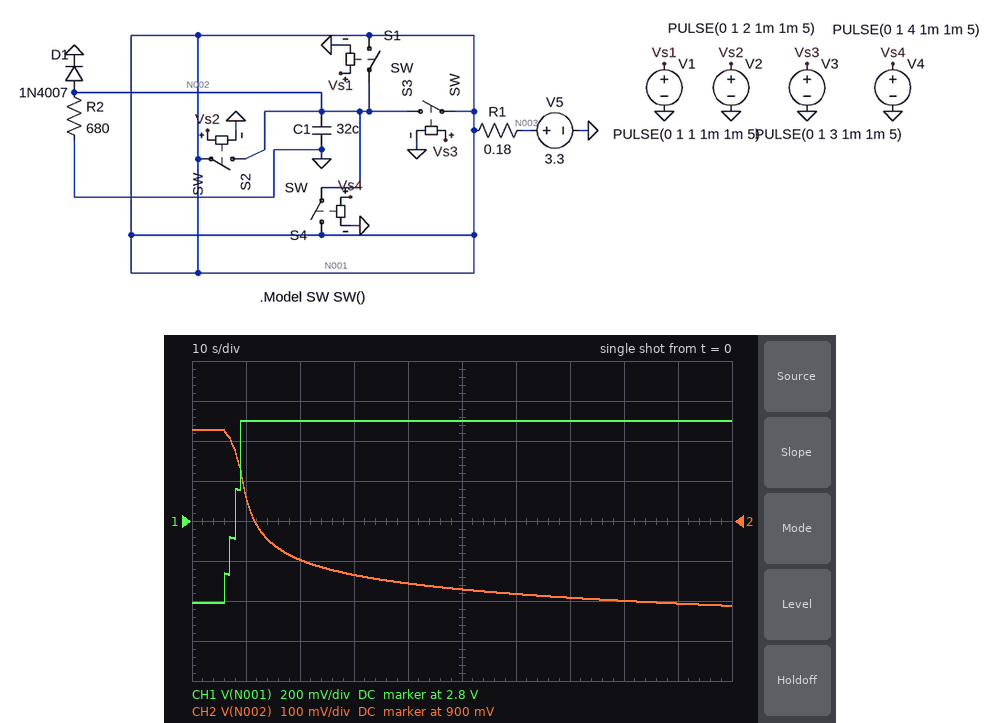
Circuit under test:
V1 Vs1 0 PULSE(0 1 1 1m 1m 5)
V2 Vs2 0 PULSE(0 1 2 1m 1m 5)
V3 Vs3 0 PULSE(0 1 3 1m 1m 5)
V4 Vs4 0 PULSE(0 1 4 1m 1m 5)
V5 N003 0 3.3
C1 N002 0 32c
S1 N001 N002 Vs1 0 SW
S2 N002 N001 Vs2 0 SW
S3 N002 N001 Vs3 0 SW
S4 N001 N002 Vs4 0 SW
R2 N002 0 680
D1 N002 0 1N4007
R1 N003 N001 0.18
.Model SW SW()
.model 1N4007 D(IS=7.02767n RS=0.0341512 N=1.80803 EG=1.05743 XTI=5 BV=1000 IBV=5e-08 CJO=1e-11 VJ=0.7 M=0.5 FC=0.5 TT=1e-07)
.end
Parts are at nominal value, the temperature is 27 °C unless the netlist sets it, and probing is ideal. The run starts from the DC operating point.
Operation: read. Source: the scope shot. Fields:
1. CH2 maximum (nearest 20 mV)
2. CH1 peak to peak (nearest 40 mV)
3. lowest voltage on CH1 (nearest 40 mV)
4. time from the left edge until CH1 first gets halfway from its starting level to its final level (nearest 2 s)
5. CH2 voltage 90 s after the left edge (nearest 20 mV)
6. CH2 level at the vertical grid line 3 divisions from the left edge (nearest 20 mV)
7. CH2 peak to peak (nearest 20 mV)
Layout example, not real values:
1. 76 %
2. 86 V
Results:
1. 1.12 V
2. 920 mV
3. 2.40 V
4. 8 s
5. 700 mV
6. 760 mV
7. 440 mV
